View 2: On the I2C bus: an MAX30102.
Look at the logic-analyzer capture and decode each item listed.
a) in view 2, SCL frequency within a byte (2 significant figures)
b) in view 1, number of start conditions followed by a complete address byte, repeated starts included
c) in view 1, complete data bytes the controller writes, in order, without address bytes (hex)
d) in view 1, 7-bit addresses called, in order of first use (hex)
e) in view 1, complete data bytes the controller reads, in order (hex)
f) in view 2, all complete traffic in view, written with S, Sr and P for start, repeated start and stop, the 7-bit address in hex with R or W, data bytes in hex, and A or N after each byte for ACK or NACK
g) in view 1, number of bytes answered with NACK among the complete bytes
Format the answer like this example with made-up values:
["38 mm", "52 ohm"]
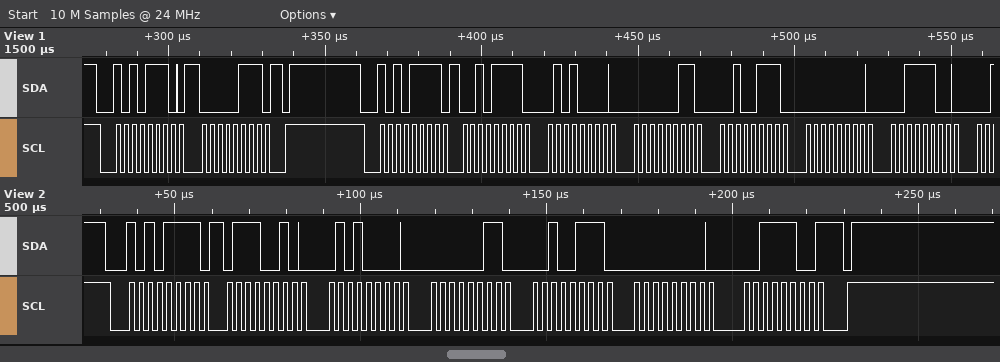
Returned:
["400 kHz", "2", "07", "0x57", "2F 50 03 27 00 3C", "S 57R A 72 A 50 A 03 A 27 A 00 A 3C N P", "0"]
